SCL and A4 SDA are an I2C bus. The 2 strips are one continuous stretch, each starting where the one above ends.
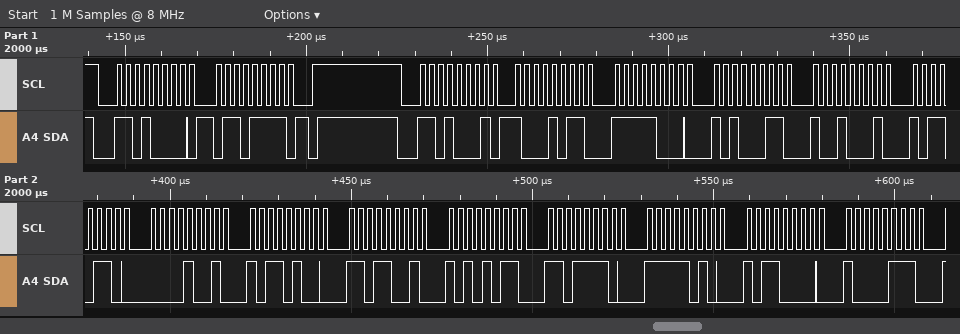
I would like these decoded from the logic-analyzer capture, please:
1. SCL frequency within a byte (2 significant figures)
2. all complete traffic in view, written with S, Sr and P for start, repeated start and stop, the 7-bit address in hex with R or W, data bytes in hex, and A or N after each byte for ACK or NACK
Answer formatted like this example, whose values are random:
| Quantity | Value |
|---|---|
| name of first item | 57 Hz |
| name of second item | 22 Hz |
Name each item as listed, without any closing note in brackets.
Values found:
| Quantity | Value |
|---|---|
| SCL frequency within a byte | 400 kHz |
| all complete traffic in view, written with S, Sr and P for start, repeated start and stop, the 7-bit address in hex with R or W, data bytes in hex, and A or N after each byte for ACK or NACK | S 68W A 6F A P S 68R A 8B A F8 A A3 A 91 A B6 A 09 A B4 A D9 A AB A DE A FA A B0 A 87 A |
